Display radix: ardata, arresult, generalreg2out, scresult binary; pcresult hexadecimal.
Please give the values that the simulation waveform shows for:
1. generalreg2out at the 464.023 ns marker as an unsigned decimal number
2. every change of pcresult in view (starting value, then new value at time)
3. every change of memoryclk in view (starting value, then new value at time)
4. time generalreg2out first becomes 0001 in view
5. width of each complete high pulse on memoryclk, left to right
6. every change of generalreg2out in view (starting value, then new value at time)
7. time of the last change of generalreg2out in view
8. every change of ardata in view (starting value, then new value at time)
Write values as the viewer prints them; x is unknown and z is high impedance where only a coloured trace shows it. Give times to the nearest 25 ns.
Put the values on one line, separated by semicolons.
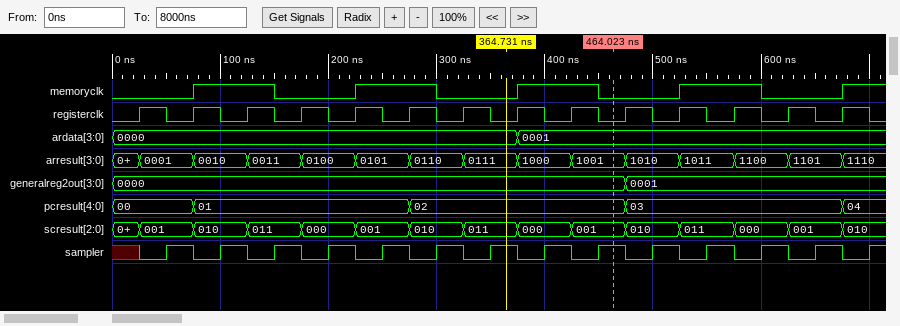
0; 00, 01 at 75 ns, 02 at 275 ns, 03 at 475 ns, 04 at 675 ns; 0, 1 at 75 ns, 0 at 150 ns, 1 at 225 ns, 0 at 300 ns, 1 at 375 ns, 0 at 450 ns, 1 at 525 ns, 0 at 600 ns, 1 at 675 ns; 475 ns; 75 ns, 75 ns, 75 ns, 75 ns; 0000, 0001 at 475 ns; 475 ns; 0000, 0001 at 375 ns
